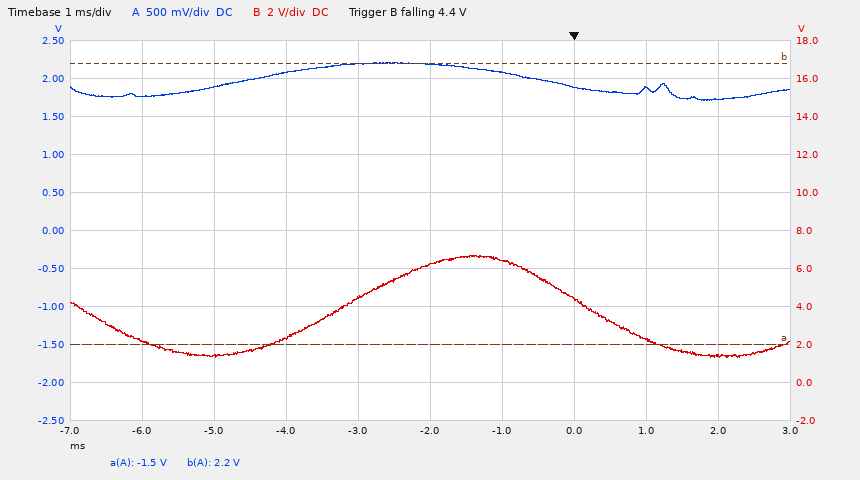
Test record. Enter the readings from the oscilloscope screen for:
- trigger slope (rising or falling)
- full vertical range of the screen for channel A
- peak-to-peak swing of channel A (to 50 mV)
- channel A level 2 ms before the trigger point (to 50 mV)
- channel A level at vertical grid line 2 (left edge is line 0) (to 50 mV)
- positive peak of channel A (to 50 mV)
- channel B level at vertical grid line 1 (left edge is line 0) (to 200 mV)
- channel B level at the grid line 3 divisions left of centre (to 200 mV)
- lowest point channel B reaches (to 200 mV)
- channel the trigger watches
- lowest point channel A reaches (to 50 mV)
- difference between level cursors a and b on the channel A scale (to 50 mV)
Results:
falling
5 V
500 mV
2.20 V
1.90 V
2.20 V
2.2 V
1.4 V
1.4 V
channel B
1.70 V
3.70 V
